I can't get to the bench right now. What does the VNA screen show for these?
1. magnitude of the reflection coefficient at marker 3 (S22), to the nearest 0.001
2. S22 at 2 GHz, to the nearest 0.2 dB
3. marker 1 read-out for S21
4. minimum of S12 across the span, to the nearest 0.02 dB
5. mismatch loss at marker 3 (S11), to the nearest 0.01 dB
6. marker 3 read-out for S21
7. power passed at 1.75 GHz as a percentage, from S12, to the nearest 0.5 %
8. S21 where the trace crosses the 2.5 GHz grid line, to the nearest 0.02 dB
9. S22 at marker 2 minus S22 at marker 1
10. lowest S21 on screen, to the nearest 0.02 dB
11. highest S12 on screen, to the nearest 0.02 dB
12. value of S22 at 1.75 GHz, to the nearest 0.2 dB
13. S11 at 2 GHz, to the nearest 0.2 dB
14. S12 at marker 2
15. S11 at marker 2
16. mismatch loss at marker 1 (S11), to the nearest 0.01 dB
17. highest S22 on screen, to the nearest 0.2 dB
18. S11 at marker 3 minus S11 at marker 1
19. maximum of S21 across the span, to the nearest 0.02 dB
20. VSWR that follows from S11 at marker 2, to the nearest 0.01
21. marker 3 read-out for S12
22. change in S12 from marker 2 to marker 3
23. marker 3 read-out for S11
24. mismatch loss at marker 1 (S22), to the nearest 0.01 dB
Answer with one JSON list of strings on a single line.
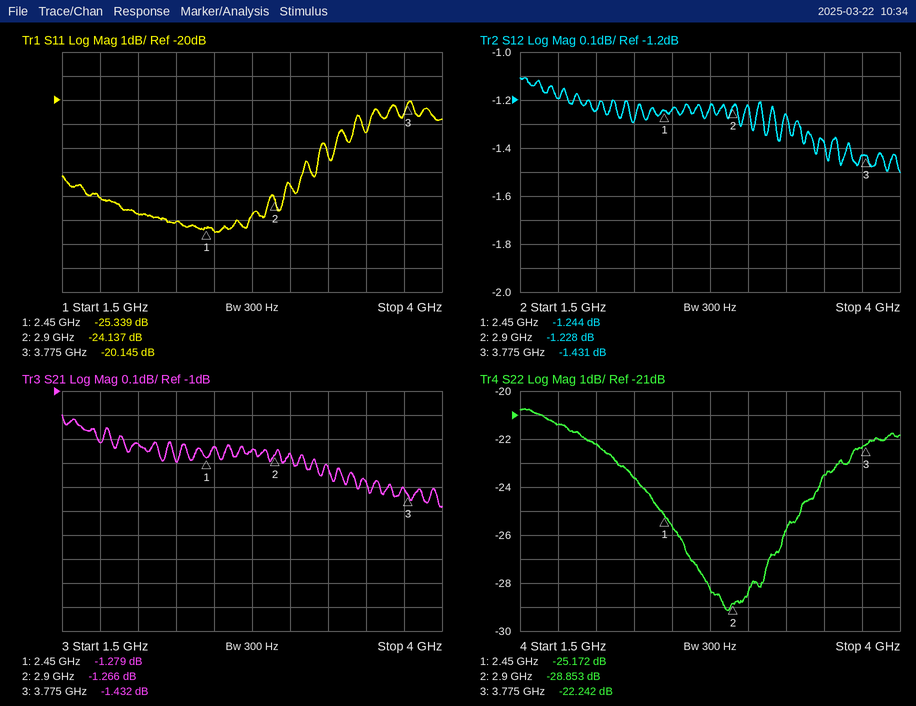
["0.077", "-22.2 dB", "-1.279 dB", "-1.50 dB", "0.04 dB", "-1.432 dB", "76.0 %", "-1.24 dB", "-3.681 dB", "-1.48 dB", "-1.10 dB", "-21.4 dB", "-24.8 dB", "-1.228 dB", "-24.137 dB", "0.01 dB", "-20.8 dB", "5.194 dB", "-1.10 dB", "1.13", "-1.431 dB", "-0.203 dB", "-20.145 dB", "0.01 dB"]
